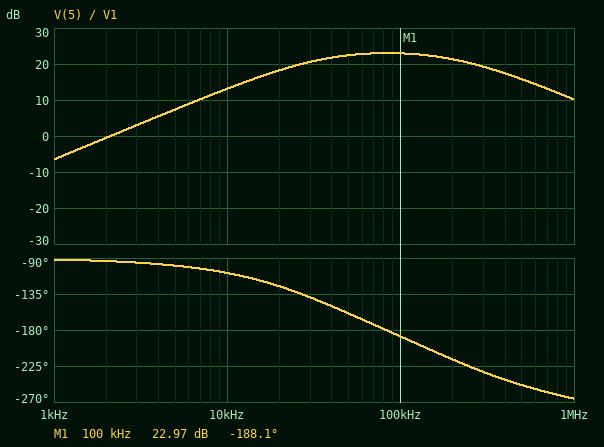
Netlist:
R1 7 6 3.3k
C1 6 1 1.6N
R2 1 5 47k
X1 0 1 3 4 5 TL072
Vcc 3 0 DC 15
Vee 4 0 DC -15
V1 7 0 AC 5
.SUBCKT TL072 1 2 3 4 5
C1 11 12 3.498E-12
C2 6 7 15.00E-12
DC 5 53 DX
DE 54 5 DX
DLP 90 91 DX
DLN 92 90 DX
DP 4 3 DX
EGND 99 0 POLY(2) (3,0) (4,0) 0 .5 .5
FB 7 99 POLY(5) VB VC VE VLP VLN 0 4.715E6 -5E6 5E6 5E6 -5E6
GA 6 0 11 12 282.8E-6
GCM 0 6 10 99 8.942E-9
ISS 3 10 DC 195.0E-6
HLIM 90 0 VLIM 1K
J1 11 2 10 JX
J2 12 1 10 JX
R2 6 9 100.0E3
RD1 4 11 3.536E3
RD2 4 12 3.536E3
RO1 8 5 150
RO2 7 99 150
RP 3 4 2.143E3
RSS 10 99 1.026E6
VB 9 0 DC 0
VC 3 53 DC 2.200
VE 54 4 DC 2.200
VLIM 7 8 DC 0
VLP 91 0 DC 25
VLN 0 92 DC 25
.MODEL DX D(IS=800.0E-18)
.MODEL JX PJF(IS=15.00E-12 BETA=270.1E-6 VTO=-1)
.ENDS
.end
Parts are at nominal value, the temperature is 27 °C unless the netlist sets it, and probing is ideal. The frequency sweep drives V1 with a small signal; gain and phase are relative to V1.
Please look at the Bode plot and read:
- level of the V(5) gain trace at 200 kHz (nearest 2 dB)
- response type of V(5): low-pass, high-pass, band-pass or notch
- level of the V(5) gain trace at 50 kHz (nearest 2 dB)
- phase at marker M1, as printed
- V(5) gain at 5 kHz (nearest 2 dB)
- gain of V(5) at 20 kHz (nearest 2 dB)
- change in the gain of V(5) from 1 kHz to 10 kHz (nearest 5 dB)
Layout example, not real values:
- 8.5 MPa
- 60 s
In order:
- 22 dB
- band-pass
- 22 dB
- -188.1 deg
- 8 dB
- 18 dB
- 20 dB
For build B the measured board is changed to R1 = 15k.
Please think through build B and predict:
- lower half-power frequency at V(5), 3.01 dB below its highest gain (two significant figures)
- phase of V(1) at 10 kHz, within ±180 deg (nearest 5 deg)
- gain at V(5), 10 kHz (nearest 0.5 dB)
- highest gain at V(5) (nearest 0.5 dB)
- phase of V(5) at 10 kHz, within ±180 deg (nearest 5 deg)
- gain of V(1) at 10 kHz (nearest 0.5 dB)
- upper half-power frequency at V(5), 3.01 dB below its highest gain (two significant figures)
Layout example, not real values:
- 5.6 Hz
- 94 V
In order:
- 6.6 kHz
- 125 deg
- 8.5 dB
- 10.0 dB
- -145 deg
- -42.5 dB
- 960 kHz
